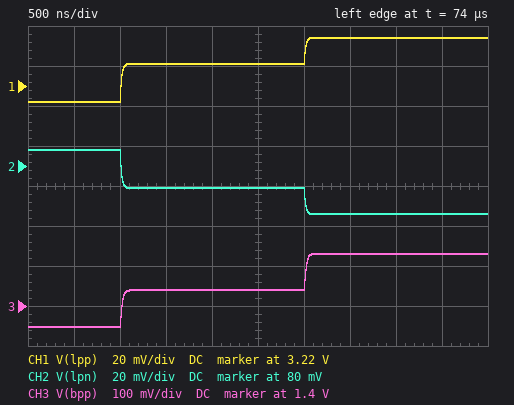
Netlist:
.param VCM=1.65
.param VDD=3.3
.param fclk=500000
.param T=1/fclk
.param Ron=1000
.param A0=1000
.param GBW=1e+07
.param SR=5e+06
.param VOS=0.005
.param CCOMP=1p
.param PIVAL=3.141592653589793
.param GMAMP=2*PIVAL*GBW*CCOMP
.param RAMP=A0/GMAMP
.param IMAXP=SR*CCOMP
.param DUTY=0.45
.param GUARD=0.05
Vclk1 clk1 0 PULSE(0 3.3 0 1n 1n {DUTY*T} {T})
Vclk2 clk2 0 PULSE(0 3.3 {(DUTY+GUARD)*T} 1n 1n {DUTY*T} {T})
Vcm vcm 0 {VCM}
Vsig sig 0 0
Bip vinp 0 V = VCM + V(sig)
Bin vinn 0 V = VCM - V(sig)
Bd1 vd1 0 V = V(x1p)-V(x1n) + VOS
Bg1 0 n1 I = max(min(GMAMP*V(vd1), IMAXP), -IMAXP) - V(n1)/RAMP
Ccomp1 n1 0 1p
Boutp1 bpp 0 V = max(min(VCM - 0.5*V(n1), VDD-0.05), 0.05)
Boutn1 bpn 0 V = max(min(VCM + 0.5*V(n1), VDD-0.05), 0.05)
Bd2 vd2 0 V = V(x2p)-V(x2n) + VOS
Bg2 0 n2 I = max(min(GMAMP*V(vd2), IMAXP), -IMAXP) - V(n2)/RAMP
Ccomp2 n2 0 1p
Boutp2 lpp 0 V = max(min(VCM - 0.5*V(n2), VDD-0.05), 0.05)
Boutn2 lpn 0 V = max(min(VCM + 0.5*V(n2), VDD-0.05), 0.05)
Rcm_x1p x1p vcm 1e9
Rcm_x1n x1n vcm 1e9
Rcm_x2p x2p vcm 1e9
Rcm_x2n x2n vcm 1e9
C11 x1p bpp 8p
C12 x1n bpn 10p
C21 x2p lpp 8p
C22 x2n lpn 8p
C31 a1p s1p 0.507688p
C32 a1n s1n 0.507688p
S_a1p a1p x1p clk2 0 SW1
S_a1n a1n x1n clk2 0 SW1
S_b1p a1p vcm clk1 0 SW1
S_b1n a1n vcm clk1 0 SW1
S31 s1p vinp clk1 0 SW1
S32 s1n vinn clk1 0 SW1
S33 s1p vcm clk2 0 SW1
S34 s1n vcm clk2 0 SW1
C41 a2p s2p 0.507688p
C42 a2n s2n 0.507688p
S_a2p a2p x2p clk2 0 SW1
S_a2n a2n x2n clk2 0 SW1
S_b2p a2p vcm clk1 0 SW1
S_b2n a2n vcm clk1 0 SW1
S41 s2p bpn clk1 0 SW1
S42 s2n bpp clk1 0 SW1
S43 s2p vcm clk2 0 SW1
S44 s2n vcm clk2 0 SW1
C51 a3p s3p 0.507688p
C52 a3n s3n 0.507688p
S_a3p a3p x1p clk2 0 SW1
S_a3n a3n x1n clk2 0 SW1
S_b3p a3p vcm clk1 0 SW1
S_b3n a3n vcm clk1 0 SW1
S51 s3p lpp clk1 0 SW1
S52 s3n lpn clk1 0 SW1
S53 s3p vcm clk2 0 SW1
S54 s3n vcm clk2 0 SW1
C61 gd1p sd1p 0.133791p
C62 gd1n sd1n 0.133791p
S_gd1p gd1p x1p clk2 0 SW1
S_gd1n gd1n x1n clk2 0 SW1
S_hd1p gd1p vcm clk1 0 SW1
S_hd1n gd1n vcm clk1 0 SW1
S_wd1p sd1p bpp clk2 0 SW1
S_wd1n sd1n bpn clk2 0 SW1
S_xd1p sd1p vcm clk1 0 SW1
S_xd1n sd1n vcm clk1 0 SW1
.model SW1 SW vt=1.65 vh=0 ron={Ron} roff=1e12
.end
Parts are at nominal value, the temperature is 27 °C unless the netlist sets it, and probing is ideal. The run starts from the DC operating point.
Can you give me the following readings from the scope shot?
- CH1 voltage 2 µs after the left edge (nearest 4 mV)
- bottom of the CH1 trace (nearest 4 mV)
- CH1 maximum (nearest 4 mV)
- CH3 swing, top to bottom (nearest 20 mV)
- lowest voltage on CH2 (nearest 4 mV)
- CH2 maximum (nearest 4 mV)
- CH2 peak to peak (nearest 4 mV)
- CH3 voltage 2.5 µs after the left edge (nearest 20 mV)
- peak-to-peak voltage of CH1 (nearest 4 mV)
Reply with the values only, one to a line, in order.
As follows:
3.232 V
3.212 V
3.244 V
180 mV
56 mV
88 mV
32 mV
1.44 V
32 mV
